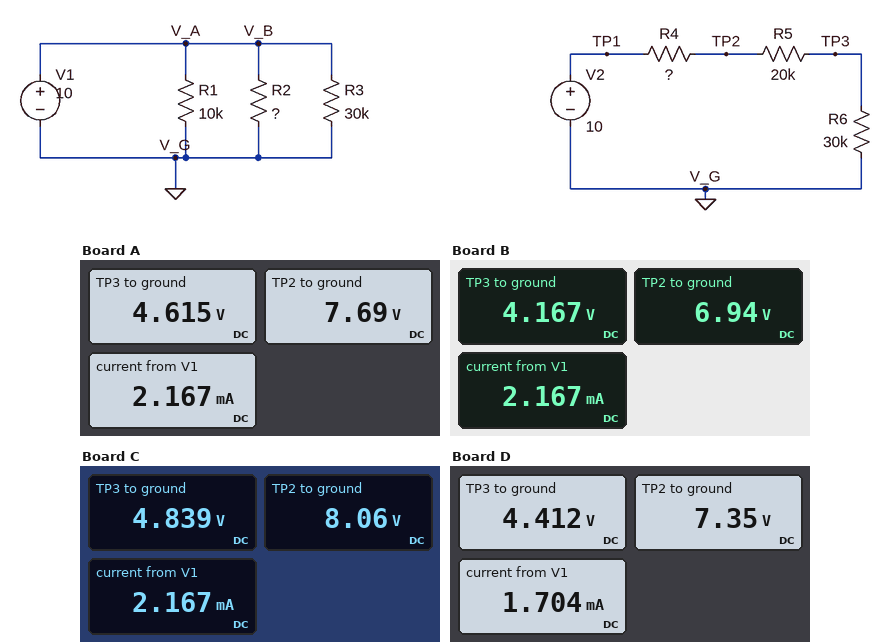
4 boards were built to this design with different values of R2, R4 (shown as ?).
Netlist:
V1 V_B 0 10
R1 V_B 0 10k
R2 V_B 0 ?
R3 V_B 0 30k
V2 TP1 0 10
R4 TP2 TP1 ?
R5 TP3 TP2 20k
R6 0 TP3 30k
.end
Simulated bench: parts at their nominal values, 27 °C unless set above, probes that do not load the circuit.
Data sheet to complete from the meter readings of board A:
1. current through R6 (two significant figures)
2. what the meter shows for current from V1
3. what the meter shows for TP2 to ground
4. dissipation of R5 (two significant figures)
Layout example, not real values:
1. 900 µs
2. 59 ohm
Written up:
1. 150 µA
2. 2.167 mA
3. 7.69 V
4. 470 µW
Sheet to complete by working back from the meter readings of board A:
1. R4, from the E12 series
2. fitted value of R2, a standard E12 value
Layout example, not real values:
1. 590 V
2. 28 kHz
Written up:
1. 15 kΩ
2. 12 kΩ
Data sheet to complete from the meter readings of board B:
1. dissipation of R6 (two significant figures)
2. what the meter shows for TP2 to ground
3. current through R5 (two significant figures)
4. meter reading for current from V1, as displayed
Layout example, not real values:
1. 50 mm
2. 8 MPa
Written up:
1. 580 µW
2. 6.94 V
3. 140 µA
4. 2.167 mA
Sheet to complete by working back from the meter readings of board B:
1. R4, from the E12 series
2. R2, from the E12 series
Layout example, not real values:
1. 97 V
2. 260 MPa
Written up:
1. 22 kΩ
2. 12 kΩ
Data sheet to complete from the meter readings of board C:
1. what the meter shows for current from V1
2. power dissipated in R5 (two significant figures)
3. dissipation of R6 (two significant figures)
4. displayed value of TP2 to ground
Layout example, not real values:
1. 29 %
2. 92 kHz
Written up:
1. 2.167 mA
2. 520 µW
3. 780 µW
4. 8.06 V
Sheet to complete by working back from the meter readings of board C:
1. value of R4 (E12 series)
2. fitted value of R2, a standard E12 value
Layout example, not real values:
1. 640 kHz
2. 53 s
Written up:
1. 12 kΩ
2. 12 kΩ
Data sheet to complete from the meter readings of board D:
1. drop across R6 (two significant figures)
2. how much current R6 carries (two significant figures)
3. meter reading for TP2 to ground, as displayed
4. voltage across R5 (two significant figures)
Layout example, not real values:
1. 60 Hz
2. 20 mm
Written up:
1. 4.4 V
2. 150 µA
3. 7.35 V
4. 2.9 V
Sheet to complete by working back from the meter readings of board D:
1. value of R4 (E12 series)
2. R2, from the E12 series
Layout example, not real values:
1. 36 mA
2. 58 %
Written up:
1. 18 kΩ
2. 27 kΩ
